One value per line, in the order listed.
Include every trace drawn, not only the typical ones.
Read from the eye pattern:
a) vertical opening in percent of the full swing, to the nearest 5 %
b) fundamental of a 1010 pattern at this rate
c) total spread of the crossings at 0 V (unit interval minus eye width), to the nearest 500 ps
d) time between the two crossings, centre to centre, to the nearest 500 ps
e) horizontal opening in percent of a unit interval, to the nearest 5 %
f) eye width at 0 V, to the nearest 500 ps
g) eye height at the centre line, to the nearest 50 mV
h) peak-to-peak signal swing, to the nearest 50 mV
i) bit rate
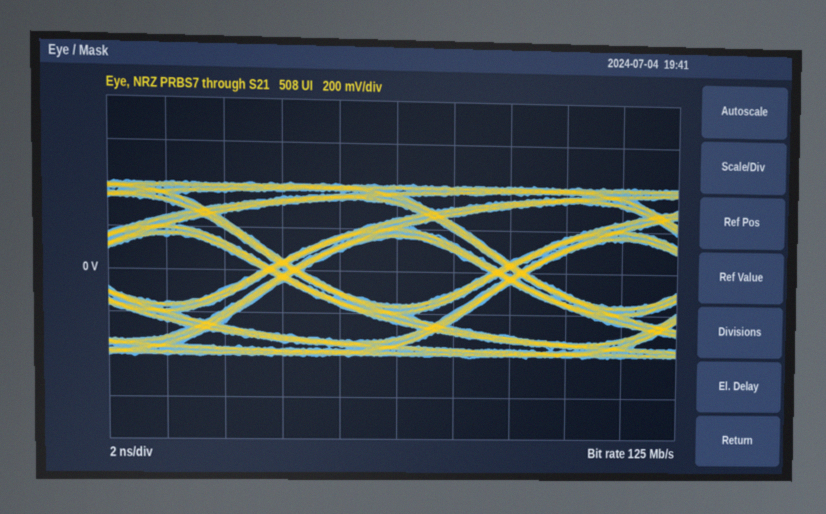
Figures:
40 %
62.5 MHz
1.5 ns
8.0 ns
80 %
6.5 ns
300 mV
800 mV
125 Mb/s
